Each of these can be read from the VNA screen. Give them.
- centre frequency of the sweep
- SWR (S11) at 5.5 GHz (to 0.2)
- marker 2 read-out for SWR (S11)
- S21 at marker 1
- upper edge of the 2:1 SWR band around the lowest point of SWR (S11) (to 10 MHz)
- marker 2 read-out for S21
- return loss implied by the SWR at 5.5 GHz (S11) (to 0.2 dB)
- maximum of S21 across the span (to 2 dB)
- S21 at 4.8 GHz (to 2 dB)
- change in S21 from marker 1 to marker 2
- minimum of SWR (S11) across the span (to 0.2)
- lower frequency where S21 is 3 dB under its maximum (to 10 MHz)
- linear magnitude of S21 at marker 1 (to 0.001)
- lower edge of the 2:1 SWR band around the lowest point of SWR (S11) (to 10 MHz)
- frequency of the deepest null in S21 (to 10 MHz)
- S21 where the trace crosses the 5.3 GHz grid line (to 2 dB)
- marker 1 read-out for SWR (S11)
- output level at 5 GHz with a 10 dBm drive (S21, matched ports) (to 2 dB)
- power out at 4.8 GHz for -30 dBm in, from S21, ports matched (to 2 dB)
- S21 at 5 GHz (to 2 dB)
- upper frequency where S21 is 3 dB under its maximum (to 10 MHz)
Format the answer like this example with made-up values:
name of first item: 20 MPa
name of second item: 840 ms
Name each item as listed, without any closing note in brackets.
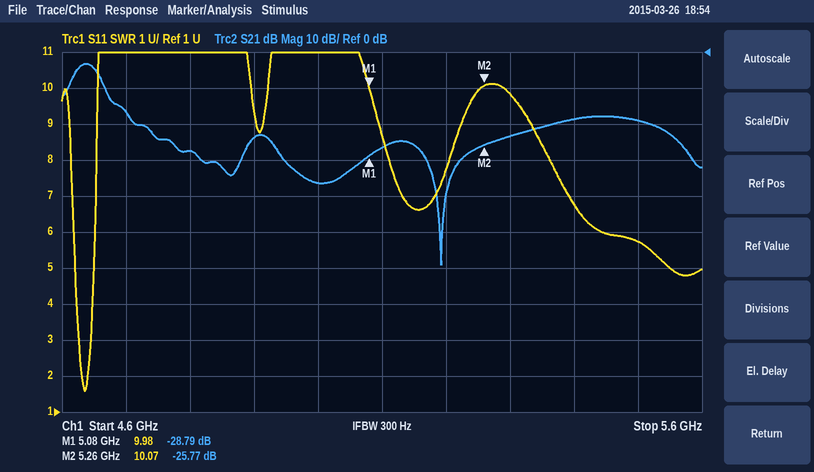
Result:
centre frequency of the sweep: 5.1 GHz
SWR (S11) at 5.5 GHz: 5.8
marker 2 read-out for SWR: 10.07
S21 at marker 1: -28.79 dB
upper edge of the 2:1 SWR band around the lowest point of SWR (S11): 4.64 GHz
marker 2 read-out for S21: -25.77 dB
return loss implied by the SWR at 5.5 GHz (S11): 3.0 dB
maximum of S21 across the span: -4 dB
S21 at 4.8 GHz: -28 dB
change in S21 from marker 1 to marker 2: 3.02 dB
minimum of SWR (S11) across the span: 1.6
lower frequency where S21 is 3 dB under its maximum: 4.62 GHz
linear magnitude of S21 at marker 1: 0.036
lower edge of the 2:1 SWR band around the lowest point of SWR (S11): 4.63 GHz
frequency of the deepest null in S21: 5.19 GHz
S21 where the trace crosses the 5.3 GHz grid line: -24 dB
marker 1 read-out for SWR: 9.98
output level at 5 GHz with a 10 dBm drive (S21, matched ports): -26 dBm
power out at 4.8 GHz for -30 dBm in, from S21, ports matched: -58 dBm
S21 at 5 GHz: -36 dB
upper frequency where S21 is 3 dB under its maximum: 4.66 GHz
